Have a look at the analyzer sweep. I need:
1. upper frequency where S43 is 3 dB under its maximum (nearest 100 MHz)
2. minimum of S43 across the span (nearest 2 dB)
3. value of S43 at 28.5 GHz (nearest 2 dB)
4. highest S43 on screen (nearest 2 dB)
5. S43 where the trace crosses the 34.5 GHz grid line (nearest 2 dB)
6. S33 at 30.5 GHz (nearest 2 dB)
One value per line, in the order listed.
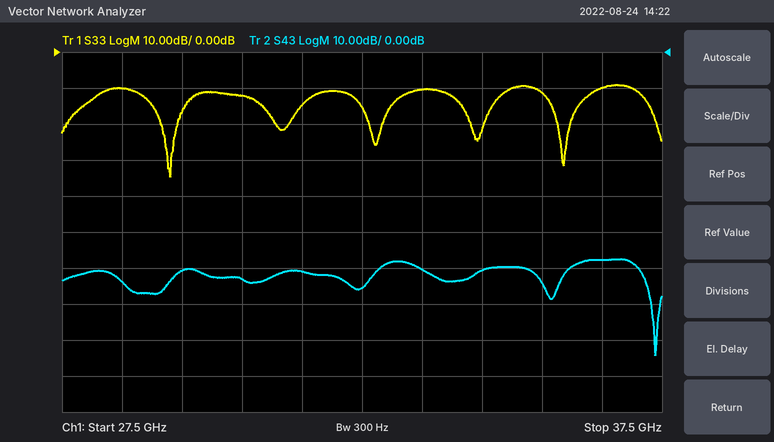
37.1 GHz
-84 dB
-64 dB
-58 dB
-60 dB
-12 dB
